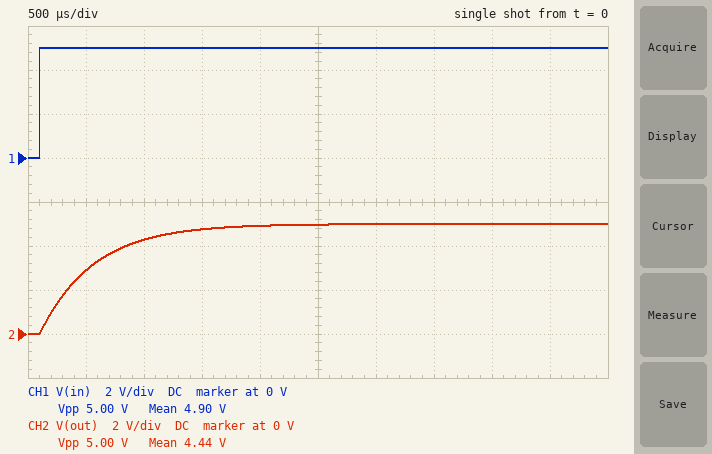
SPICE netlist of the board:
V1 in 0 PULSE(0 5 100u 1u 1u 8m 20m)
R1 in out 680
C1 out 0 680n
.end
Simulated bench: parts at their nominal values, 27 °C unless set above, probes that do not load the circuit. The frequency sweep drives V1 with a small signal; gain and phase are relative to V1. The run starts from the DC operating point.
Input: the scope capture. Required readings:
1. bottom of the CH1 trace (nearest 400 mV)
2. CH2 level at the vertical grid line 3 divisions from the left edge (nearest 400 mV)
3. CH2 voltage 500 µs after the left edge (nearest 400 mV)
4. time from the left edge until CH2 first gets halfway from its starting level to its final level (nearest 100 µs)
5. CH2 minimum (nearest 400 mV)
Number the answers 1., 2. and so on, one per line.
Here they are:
1. 0 V
2. 4.8 V
3. 2.8 V
4. 400 µs
5. 0 V
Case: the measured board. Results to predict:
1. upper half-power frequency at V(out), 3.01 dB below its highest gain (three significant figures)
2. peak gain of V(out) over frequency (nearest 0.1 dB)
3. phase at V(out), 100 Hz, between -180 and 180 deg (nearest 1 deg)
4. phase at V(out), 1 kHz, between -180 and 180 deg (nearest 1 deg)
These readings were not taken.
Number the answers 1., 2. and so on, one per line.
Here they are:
1. 344 Hz
2. 0 dB
3. -16 deg
4. -71 deg
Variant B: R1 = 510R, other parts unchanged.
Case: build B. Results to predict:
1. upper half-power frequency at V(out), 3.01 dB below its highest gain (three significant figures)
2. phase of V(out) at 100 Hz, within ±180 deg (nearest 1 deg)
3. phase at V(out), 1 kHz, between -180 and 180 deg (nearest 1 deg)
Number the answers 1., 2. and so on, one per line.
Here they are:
1. 459 Hz
2. -12 deg
3. -65 deg
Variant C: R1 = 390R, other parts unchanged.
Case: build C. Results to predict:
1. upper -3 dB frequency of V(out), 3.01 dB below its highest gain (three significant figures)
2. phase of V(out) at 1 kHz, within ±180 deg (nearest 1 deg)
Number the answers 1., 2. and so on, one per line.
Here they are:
1. 600 Hz
2. -59 deg
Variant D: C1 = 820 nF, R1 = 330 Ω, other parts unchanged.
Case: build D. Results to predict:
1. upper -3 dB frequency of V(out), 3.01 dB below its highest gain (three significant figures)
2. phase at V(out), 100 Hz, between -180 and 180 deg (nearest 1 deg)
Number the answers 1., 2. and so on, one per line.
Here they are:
1. 588 Hz
2. -10 deg
